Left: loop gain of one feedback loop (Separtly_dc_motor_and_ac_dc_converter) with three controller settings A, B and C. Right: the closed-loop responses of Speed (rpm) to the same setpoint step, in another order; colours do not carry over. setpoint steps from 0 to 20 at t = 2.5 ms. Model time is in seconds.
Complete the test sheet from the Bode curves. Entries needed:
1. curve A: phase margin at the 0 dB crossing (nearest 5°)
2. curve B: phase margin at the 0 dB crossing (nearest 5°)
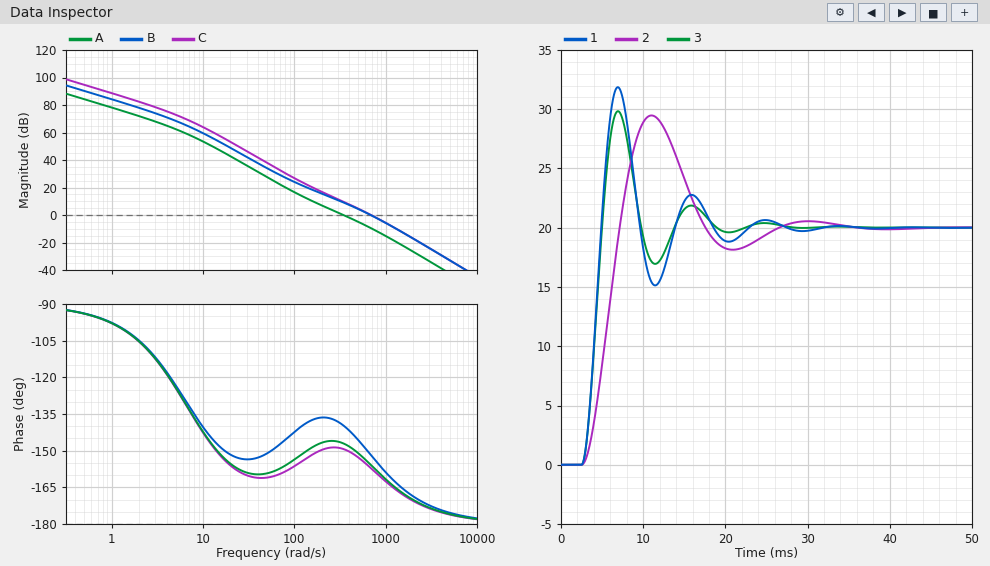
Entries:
35°
30°
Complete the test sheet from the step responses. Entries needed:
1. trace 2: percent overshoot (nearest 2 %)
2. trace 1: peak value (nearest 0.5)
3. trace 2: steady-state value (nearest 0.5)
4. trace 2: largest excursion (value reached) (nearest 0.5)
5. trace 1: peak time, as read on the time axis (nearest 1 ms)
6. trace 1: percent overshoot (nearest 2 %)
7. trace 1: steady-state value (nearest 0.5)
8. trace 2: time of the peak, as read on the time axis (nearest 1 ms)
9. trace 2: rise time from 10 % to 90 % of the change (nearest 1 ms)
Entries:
48 %
32.0
20.0
29.5
7 ms
60 %
20.0
11 ms
3 ms
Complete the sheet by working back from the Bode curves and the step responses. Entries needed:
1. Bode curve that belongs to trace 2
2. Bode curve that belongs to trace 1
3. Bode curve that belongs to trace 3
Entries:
A
C
B
